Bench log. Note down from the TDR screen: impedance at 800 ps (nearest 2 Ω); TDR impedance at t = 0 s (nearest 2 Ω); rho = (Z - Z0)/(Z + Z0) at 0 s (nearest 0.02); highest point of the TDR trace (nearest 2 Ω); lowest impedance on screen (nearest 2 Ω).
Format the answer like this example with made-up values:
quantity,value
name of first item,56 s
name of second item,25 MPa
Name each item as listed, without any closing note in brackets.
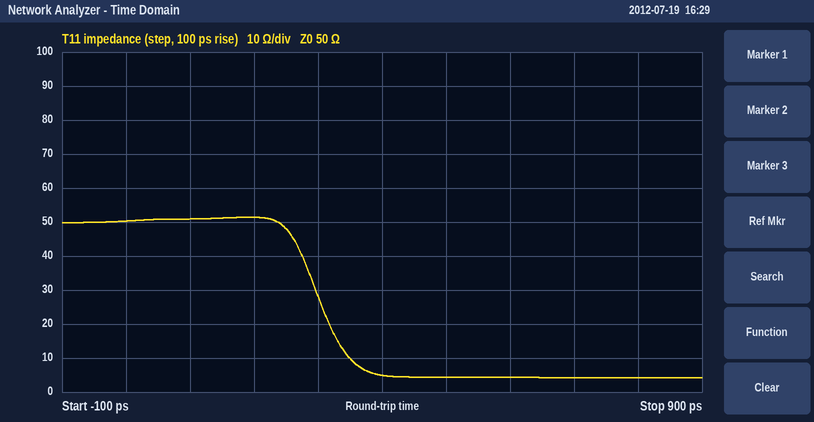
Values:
quantity,value
impedance at 800 ps,4 Ω
TDR impedance at t = 0 s,50 Ω
rho = (Z - Z0)/(Z + Z0) at 0 s,0.00
highest point of the TDR trace,52 Ω
lowest impedance on screen,4 Ω
